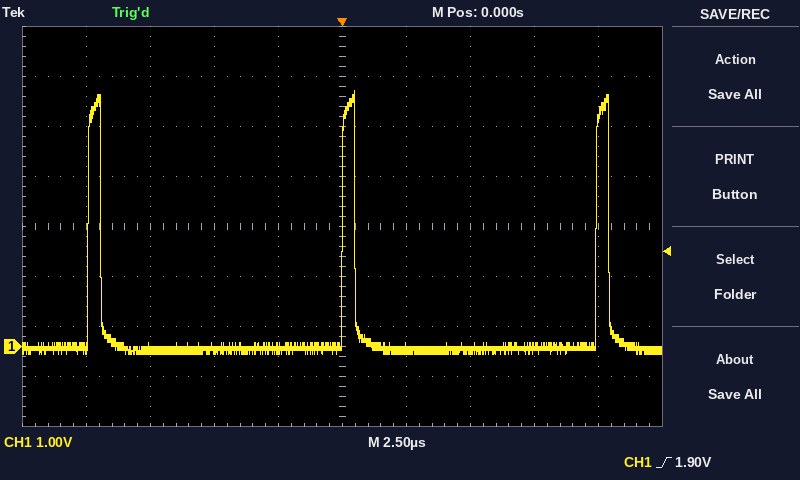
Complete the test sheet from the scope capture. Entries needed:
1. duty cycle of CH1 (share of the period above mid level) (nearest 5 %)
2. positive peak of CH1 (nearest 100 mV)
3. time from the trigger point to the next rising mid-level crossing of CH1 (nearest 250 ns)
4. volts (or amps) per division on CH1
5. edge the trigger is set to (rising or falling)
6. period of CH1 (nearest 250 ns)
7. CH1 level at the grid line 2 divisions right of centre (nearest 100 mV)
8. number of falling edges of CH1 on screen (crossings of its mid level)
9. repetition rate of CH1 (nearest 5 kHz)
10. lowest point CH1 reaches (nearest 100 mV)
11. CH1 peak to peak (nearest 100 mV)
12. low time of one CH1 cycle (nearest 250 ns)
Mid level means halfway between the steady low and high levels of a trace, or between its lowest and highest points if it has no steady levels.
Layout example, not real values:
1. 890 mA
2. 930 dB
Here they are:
1. 5 %
2. 5.1 V
3. 10.00 µs
4. 1 V
5. rising
6. 10.00 µs
7. -100 mV
8. 3
9. 100 kHz
10. -200 mV
11. 5.3 V
12. 9.50 µs
